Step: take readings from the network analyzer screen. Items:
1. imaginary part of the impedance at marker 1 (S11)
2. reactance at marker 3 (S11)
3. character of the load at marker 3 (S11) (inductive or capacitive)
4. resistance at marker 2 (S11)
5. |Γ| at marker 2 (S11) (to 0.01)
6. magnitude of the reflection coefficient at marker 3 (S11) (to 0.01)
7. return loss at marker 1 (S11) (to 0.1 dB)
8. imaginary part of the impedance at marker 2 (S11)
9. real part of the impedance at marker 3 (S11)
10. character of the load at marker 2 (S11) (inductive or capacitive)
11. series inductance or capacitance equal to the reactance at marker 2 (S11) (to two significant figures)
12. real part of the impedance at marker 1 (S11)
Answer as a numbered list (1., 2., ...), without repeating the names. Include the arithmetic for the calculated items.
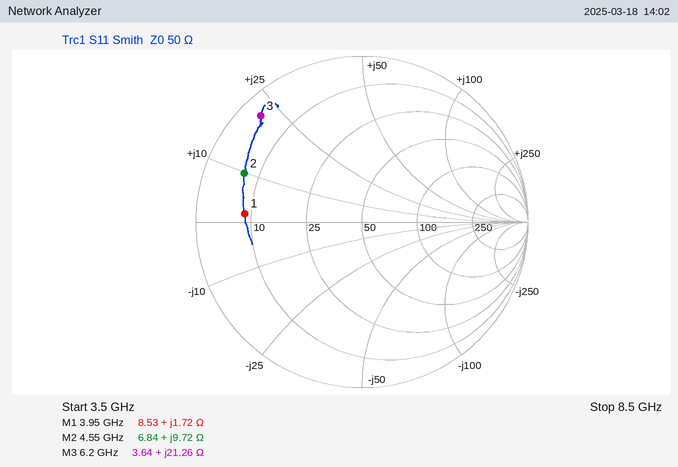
1. +1.72 Ω
2. +21.26 Ω
3. inductive
4. 6.84 Ω
5. 0.77
6. 0.88
7. 3.0 dB
8. +9.72 Ω
9. 3.64 Ω
10. inductive
11. L = 9.72 Ω/(2π × 4.55 GHz) ≈ 340 pH
12. 8.53 Ω
